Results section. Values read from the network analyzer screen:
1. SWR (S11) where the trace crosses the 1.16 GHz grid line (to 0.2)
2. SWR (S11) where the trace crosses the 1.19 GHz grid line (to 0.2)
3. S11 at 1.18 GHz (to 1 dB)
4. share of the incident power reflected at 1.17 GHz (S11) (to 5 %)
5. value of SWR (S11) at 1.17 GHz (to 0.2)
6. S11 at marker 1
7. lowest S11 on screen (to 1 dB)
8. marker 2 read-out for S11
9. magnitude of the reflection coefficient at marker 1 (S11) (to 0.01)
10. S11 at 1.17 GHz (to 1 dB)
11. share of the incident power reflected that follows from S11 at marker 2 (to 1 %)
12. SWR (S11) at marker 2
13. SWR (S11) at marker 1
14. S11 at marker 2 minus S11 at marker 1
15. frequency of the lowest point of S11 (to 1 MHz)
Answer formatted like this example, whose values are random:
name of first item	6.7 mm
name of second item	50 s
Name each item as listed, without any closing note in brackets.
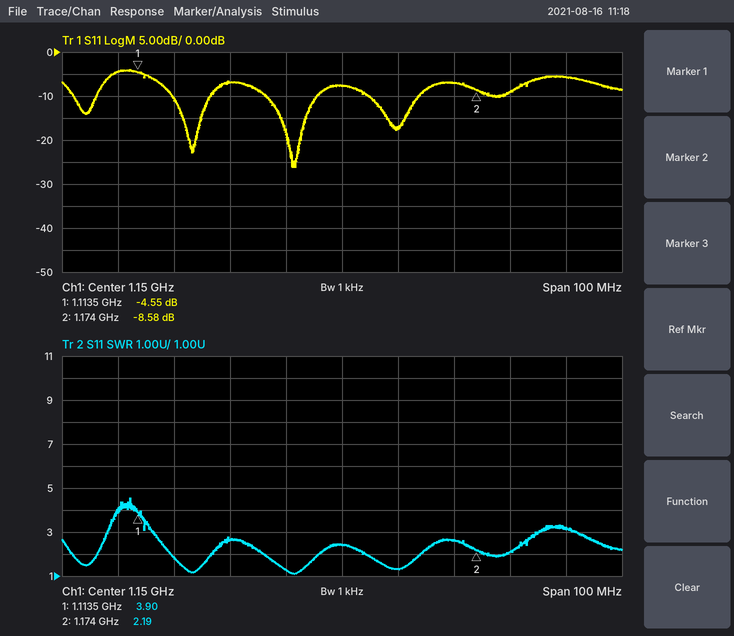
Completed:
SWR (S11) where the trace crosses the 1.16 GHz grid line	1.4
SWR (S11) where the trace crosses the 1.19 GHz grid line	3.2
S11 at 1.18 GHz	-9 dB
share of the incident power reflected at 1.17 GHz (S11)	20 %
value of SWR (S11) at 1.17 GHz	2.6
S11 at marker 1	-4.55 dB
lowest S11 on screen	-26 dB
marker 2 read-out for S11	-8.58 dB
magnitude of the reflection coefficient at marker 1 (S11)	0.59
S11 at 1.17 GHz	-7 dB
share of the incident power reflected that follows from S11 at marker 2	14 %
SWR (S11) at marker 2	2.19
SWR (S11) at marker 1	3.90
S11 at marker 2 minus S11 at marker 1	-4.03 dB
frequency of the lowest point of S11	1.141 GHz
